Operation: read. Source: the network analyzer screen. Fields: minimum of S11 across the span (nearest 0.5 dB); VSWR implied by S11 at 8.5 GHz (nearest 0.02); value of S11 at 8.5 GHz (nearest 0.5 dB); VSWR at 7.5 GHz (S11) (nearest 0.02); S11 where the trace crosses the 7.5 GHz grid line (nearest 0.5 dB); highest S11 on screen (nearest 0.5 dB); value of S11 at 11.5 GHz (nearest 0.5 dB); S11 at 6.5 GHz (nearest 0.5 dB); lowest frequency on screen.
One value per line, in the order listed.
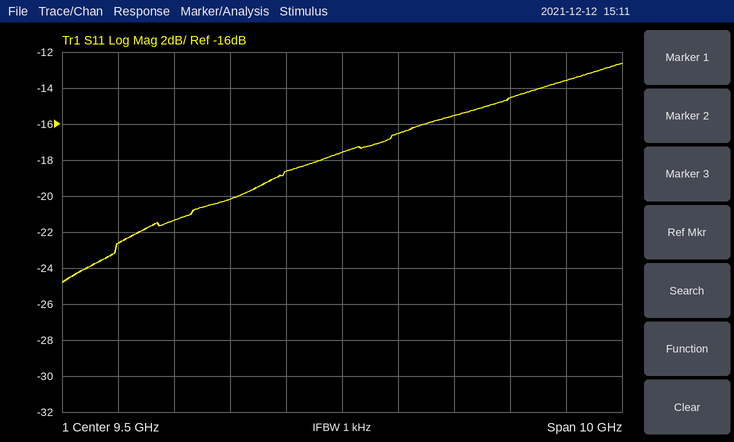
-25.0 dB
1.26
-18.5 dB
1.22
-20.0 dB
-12.5 dB
-15.5 dB
-21.5 dB
4.5 GHz
